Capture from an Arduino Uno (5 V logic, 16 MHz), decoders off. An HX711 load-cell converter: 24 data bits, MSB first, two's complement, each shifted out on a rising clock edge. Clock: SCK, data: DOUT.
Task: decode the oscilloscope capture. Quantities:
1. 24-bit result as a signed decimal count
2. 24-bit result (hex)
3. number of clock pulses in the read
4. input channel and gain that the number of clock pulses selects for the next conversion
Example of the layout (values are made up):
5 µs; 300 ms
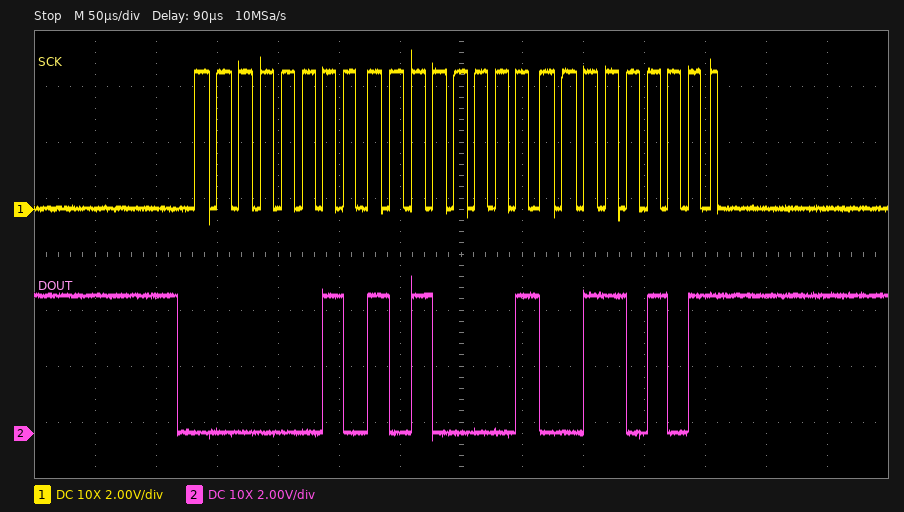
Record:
172341; 0x02A135; 25; channel A, gain 128
